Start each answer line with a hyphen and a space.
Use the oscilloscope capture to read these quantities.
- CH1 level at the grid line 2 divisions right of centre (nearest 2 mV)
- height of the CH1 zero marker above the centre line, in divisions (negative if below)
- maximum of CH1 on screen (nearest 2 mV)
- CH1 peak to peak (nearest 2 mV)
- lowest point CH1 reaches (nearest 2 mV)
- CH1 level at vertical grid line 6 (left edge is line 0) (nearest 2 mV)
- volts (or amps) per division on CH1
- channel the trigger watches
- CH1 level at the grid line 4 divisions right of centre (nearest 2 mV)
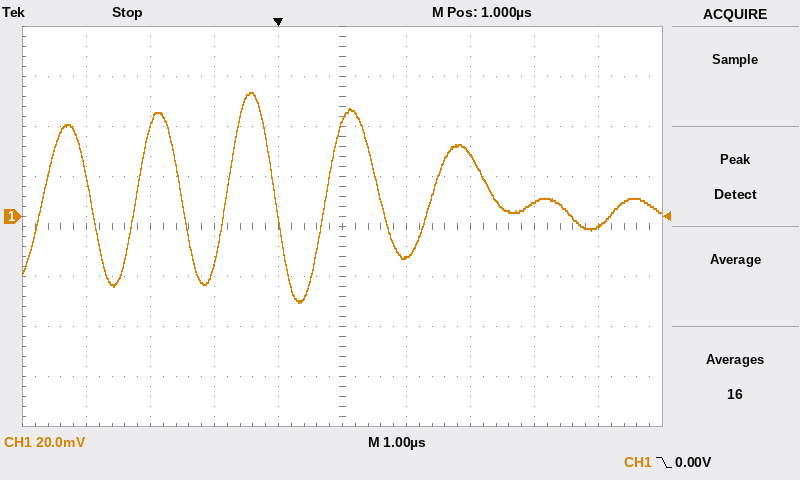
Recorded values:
- 24 mV
- +0.2 div
- 50 mV
- 84 mV
- -34 mV
- -16 mV
- 20 mV
- CH1
- -4 mV
